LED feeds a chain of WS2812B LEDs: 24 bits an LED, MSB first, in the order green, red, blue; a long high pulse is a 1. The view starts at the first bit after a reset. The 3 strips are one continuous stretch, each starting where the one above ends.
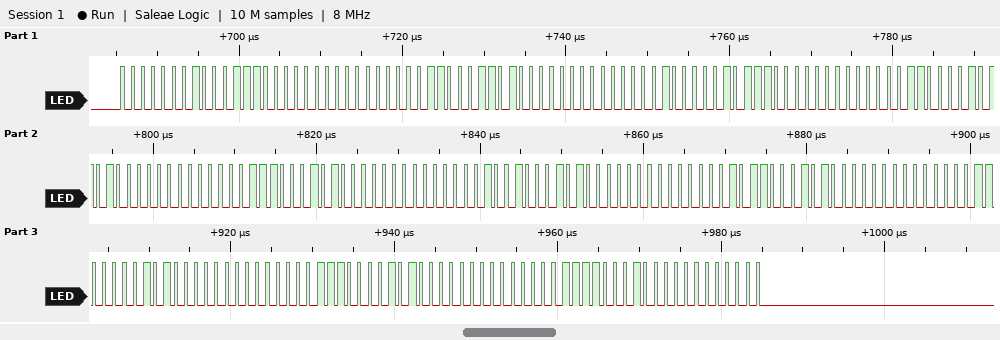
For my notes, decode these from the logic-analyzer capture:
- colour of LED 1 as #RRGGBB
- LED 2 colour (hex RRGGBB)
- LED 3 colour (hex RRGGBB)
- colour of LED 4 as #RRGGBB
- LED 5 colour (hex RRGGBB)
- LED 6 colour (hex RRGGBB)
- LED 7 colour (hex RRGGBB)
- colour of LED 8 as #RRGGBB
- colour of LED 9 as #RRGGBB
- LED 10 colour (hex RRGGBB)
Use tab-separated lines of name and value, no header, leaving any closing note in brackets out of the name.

colour of LED 1 as #RRGGBB	#1C0100
LED 2 colour	#1A0300
LED 3 colour	#170400
colour of LED 4 as #RRGGBB	#150600
LED 5 colour	#140700
LED 6 colour	#140900
LED 7 colour	#140B00
colour of LED 8 as #RRGGBB	#140C00
colour of LED 9 as #RRGGBB	#140E00
LED 10 colour	#100F00
